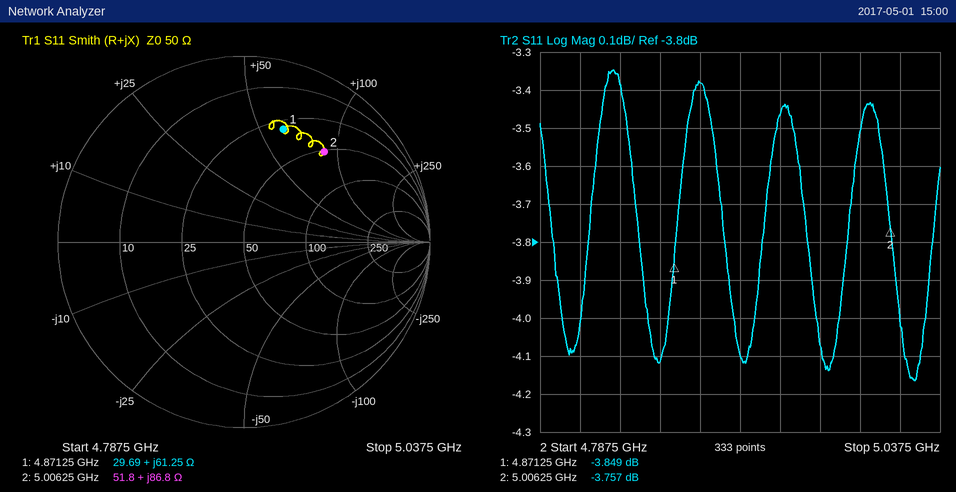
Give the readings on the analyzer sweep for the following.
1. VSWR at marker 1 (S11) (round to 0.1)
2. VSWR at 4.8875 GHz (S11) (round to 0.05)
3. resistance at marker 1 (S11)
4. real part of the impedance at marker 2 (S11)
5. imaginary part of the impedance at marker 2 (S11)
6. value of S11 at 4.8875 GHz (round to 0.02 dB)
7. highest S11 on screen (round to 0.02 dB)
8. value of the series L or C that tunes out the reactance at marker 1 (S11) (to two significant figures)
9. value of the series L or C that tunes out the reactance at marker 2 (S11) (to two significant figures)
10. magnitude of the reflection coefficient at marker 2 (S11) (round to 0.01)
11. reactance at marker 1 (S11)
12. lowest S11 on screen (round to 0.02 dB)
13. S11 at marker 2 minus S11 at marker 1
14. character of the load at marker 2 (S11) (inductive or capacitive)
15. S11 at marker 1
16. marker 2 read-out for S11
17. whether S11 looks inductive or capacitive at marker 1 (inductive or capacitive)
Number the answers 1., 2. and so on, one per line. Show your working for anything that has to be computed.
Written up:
1. (1 + 0.6420)/(1 − 0.6420) ≈ 4.6
2. |Γ| = 10^(-3.38/20) = 0.6776; VSWR = (1 + 0.6776)/(1 − 0.6776) ≈ 5.20
3. 29.69 Ω
4. 51.8 Ω
5. +86.8 Ω
6. -3.38 dB
7. -3.34 dB
8. C = 1/(2π × 4.87125 GHz × 61.25 Ω) ≈ 533 fF, so 530 fF to two significant figures
9. C = 1/(2π × 5.00625 GHz × 86.8 Ω) ≈ 366 fF, so 370 fF to two significant figures
10. 0.65
11. +61.25 Ω
12. -4.16 dB
13. -3.757 − (-3.849) = 0.092 dB
14. inductive
15. -3.849 dB
16. -3.757 dB
17. inductive
